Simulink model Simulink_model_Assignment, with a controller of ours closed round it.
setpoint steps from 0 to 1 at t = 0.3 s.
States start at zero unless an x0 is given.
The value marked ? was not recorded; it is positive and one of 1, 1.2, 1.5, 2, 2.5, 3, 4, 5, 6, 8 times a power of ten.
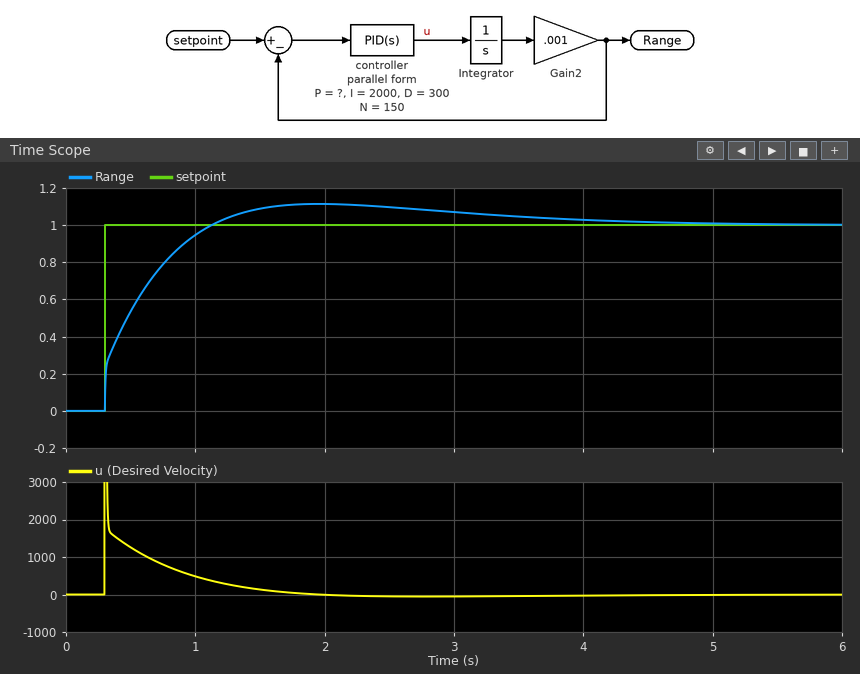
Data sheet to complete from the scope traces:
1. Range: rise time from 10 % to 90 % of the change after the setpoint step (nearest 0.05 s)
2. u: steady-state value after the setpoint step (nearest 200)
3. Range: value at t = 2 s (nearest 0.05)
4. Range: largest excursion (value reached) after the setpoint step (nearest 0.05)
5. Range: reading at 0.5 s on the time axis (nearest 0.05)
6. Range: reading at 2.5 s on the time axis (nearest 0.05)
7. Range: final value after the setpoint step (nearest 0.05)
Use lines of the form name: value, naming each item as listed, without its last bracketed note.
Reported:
Range: rise time from 10 % to 90 % of the change after the setpoint step: 0.60 s
u: steady-state value after the setpoint step: 0
Range: value at t = 2 s: 1.10
Range: largest excursion (value reached) after the setpoint step: 1.10
Range: reading at 0.5 s on the time axis: 0.55
Range: reading at 2.5 s on the time axis: 1.10
Range: final value after the setpoint step: 1.00
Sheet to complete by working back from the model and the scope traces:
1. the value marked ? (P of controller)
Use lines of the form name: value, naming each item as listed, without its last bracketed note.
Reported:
the value marked ?: 3000
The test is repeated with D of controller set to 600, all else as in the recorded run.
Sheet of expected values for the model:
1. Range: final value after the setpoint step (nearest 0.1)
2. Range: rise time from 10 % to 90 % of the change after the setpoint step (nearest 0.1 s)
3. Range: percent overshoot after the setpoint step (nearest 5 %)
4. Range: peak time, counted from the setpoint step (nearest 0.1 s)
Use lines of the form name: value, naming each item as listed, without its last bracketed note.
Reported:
Range: final value after the setpoint step: 1.0
Range: rise time from 10 % to 90 % of the change after the setpoint step: 0.7 s
Range: percent overshoot after the setpoint step: 10 %
Range: peak time, counted from the setpoint step: 1.9 s
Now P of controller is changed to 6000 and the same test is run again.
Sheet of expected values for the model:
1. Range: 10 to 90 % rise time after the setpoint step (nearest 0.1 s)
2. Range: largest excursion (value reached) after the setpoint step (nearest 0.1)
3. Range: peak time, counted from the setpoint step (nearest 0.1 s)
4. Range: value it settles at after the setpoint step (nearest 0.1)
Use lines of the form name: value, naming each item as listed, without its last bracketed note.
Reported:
Range: 10 to 90 % rise time after the setpoint step: 0.4 s
Range: largest excursion (value reached) after the setpoint step: 1.0
Range: peak time, counted from the setpoint step: 1.3 s
Range: value it settles at after the setpoint step: 1.0
